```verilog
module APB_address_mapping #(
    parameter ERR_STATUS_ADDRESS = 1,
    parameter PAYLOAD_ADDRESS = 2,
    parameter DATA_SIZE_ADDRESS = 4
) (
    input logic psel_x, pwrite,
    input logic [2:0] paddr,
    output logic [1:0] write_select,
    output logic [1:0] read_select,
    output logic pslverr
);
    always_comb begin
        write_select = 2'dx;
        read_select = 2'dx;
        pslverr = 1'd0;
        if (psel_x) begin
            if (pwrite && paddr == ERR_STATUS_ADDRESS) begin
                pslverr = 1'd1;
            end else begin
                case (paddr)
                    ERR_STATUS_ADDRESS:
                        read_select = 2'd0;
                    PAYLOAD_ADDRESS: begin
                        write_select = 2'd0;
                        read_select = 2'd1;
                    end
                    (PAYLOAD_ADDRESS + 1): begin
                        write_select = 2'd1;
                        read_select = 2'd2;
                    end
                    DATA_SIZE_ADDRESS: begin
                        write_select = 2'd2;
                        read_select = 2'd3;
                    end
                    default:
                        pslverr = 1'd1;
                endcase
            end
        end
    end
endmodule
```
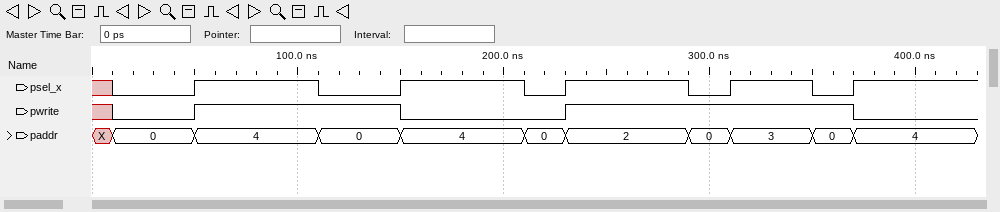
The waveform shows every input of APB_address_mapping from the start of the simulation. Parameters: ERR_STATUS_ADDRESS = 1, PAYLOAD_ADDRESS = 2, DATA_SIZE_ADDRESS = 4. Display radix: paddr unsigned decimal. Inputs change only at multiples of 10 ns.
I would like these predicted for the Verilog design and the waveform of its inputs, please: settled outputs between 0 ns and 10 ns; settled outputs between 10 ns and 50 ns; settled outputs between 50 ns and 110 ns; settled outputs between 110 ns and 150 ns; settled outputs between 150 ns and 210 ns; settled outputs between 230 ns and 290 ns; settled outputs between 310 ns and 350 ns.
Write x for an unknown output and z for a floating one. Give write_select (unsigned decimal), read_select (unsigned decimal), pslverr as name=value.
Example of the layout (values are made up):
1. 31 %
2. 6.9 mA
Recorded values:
1. write_select=x, read_select=x, pslverr=0
2. write_select=x, read_select=x, pslverr=0
3. write_select=2, read_select=3, pslverr=0
4. write_select=x, read_select=x, pslverr=0
5. write_select=2, read_select=3, pslverr=0
6. write_select=0, read_select=1, pslverr=0
7. write_select=1, read_select=2, pslverr=0
